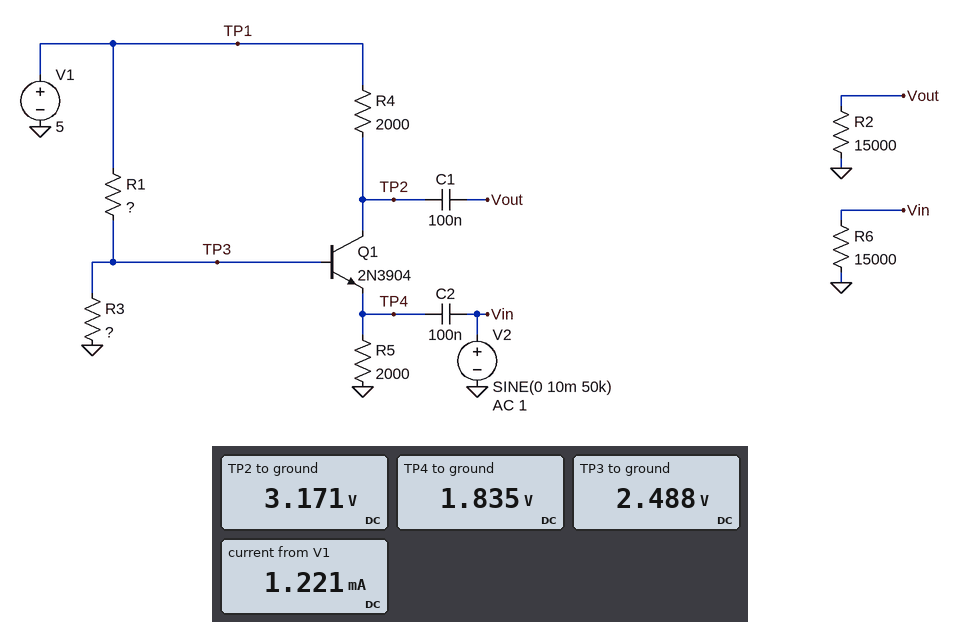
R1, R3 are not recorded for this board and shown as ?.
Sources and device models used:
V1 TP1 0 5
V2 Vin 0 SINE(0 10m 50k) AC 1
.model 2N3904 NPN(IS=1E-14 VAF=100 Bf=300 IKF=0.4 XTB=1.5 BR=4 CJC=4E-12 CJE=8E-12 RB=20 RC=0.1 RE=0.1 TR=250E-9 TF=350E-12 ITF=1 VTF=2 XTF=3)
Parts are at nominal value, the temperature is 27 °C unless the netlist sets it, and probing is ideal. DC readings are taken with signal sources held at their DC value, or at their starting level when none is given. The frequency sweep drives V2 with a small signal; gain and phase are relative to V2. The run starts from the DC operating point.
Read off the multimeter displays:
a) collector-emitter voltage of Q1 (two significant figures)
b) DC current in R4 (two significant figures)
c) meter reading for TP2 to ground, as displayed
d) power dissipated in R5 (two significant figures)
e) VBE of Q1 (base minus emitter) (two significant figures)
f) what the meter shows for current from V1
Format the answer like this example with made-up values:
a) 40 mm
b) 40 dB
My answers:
a) 1.3 V
b) 910 µA
c) 3.171 V
d) 1.7 mW
e) 650 mV
f) 1.221 mA
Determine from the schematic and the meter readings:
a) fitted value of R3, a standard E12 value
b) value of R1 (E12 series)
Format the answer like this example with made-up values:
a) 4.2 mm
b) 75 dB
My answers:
a) 8.2 kΩ
b) 8.2 kΩ
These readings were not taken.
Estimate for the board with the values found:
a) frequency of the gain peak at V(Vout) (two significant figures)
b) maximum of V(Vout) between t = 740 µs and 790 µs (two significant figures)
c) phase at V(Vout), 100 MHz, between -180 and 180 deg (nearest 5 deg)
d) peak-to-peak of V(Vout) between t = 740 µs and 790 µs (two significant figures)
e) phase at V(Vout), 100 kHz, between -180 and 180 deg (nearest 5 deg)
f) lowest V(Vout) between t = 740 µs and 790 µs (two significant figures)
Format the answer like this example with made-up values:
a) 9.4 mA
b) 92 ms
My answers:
a) 98 kHz
b) 340 mV
c) -5 deg
d) 710 mV
e) 0 deg
f) -370 mV
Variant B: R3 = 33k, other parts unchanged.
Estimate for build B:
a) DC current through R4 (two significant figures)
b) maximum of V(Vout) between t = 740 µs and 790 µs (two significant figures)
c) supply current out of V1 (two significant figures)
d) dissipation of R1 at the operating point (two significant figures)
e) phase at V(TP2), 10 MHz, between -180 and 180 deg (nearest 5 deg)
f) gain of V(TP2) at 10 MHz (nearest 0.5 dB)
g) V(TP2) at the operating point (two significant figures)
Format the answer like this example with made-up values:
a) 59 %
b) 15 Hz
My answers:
a) 1.2 mA
b) 10 mV
c) 1.4 mA
d) 370 µW
e) 0 deg
f) 0 dB
g) 2.6 V
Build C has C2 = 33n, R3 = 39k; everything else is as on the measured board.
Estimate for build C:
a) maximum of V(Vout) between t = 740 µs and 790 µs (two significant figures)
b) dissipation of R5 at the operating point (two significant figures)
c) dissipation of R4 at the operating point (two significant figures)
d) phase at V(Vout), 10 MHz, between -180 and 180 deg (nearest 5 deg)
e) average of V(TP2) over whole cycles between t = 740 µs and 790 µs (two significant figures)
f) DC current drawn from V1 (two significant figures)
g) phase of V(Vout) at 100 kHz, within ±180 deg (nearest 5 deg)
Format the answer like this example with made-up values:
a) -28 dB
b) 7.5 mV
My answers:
a) 10 mV
b) 3.4 mW
c) 2.8 mW
d) 0 deg
e) 2.6 V
f) 1.4 mA
g) 5 deg
